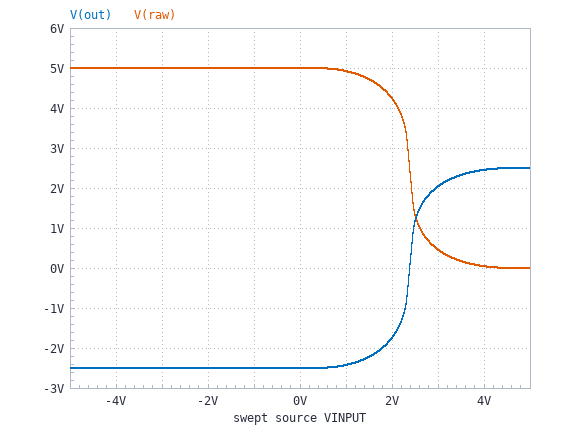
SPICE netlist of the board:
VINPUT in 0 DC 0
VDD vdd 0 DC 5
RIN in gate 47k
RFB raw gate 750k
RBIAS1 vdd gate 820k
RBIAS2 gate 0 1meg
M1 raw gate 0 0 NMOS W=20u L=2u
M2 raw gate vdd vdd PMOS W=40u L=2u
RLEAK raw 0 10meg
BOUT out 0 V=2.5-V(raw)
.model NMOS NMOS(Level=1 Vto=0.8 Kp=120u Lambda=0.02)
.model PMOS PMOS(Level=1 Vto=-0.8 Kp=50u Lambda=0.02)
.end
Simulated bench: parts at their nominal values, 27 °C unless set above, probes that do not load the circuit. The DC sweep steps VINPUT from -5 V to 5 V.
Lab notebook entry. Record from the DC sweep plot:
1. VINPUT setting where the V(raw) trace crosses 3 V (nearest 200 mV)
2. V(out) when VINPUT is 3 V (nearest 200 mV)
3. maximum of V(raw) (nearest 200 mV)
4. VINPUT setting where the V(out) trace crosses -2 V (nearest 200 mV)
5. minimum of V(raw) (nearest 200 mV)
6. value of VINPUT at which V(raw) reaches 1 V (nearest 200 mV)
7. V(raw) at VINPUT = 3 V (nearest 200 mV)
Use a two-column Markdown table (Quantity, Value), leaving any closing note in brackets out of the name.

| Quantity | Value |
|---|---|
| VINPUT setting where the V(raw) trace crosses 3 V | 2.4 V |
| V(out) when VINPUT is 3 V | 2.0 V |
| maximum of V(raw) | 5.0 V |
| VINPUT setting where the V(out) trace crosses -2 V | 1.8 V |
| minimum of V(raw) | 0 V |
| value of VINPUT at which V(raw) reaches 1 V | 2.6 V |
| V(raw) at VINPUT = 3 V | 400 mV |
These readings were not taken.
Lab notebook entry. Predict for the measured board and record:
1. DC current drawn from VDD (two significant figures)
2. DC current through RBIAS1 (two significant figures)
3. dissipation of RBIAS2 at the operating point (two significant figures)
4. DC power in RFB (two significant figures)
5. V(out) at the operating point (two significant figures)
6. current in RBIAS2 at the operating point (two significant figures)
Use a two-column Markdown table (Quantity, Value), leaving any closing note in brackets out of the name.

| Quantity | Value |
|---|---|
| DC current drawn from VDD | 12 µA |
| DC current through RBIAS1 | 5.5 µA |
| dissipation of RBIAS2 at the operating point | 260 nW |
| DC power in RFB | 27 µW |
| V(out) at the operating point | -2.5 V |
| current in RBIAS2 at the operating point | 510 nA |
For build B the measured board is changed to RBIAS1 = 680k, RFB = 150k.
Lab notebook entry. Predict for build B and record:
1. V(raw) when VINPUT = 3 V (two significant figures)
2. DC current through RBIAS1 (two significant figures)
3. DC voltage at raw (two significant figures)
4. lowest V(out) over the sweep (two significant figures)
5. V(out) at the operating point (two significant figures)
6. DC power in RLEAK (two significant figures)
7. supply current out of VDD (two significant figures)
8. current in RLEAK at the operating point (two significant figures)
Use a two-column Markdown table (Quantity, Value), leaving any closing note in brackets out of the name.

| Quantity | Value |
|---|---|
| V(raw) when VINPUT = 3 V | 950 mV |
| DC current through RBIAS1 | 5.4 µA |
| DC voltage at raw | 4.9 V |
| lowest V(out) over the sweep | -2.5 V |
| V(out) at the operating point | -2.4 V |
| DC power in RLEAK | 2.4 µW |
| supply current out of VDD | 210 µA |
| current in RLEAK at the operating point | 490 nA |
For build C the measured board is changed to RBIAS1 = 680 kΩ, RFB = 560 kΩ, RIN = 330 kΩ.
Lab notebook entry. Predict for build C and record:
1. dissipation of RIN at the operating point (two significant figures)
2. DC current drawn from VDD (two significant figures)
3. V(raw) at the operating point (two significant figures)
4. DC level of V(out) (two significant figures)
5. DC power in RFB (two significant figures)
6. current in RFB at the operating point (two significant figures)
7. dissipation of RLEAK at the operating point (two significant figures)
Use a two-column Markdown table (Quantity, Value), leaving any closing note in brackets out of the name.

| Quantity | Value |
|---|---|
| dissipation of RIN at the operating point | 13 µW |
| DC current drawn from VDD | 1.1 mA |
| V(raw) at the operating point | 4.4 V |
| DC level of V(out) | -1.9 V |
| DC power in RFB | 9.6 µW |
| current in RFB at the operating point | 4.1 µA |
| dissipation of RLEAK at the operating point | 1.9 µW |
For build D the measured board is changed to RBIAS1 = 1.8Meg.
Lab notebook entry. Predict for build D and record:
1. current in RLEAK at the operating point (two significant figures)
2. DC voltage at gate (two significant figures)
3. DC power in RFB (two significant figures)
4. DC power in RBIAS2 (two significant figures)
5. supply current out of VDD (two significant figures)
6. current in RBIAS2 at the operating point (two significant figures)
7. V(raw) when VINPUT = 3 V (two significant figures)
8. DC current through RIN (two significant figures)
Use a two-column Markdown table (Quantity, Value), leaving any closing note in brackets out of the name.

| Quantity | Value |
|---|---|
| current in RLEAK at the operating point | 500 nA |
| DC voltage at gate | 390 mV |
| DC power in RFB | 28 µW |
| DC power in RBIAS2 | 150 nW |
| supply current out of VDD | 9.2 µA |
| current in RBIAS2 at the operating point | 390 nA |
| V(raw) when VINPUT = 3 V | 520 mV |
| DC current through RIN | 8.3 µA |
